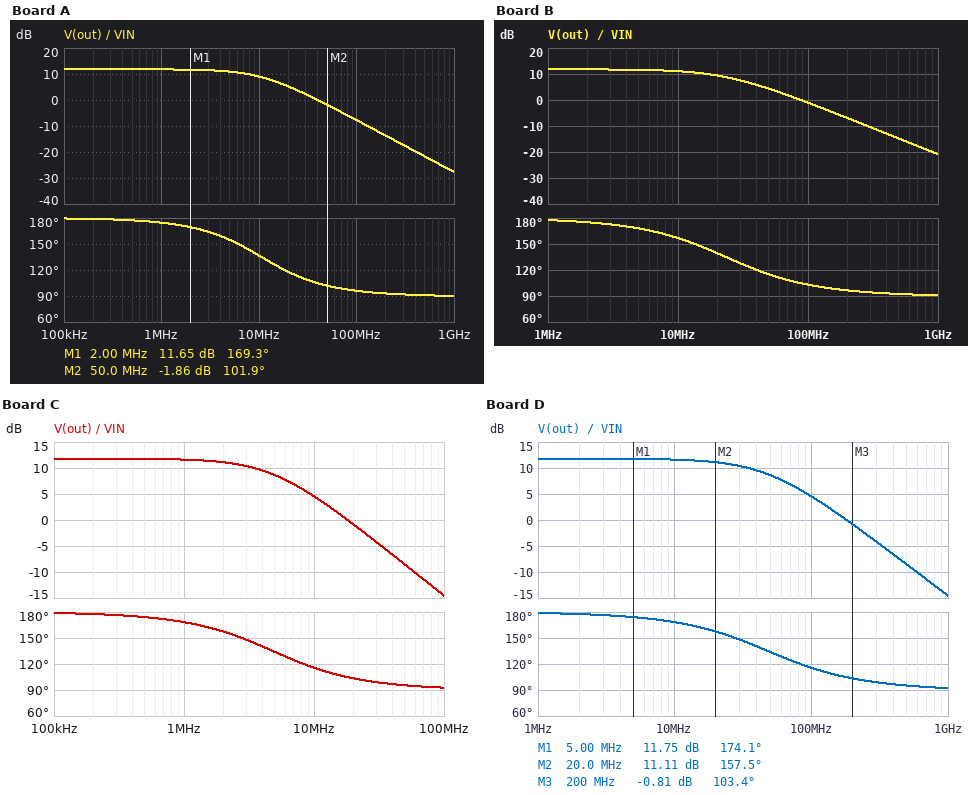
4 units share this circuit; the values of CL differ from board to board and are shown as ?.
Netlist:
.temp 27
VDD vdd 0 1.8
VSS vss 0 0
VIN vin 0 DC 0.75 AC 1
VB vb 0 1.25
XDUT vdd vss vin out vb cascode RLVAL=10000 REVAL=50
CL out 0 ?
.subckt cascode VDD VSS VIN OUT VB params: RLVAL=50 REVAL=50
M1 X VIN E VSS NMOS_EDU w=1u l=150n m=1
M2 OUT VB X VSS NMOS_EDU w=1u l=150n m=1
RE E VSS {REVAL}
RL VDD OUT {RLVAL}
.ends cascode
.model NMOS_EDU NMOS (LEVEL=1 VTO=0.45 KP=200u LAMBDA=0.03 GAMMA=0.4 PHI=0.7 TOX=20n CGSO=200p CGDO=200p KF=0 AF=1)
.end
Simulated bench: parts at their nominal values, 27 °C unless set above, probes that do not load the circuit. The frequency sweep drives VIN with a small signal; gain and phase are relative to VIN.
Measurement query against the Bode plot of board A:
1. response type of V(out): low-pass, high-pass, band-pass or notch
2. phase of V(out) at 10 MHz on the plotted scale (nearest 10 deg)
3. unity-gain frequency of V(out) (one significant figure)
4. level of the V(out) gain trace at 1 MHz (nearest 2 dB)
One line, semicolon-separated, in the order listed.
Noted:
low-pass; 140 deg; 40 MHz; 12 dB
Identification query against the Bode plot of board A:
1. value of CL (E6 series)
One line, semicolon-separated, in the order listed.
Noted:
1.5 pF
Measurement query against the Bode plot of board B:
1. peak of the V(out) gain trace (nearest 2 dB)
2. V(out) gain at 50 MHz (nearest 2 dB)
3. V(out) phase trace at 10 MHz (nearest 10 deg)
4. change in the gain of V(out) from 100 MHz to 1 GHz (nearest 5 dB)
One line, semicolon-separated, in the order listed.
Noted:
12 dB; 4 dB; 160 deg; -20 dB
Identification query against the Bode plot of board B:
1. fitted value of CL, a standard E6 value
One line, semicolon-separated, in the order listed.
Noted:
680 fF
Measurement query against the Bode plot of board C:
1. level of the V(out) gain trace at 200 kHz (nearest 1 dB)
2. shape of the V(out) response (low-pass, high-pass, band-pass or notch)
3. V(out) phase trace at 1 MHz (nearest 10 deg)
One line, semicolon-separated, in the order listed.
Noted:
12 dB; low-pass; 170 deg
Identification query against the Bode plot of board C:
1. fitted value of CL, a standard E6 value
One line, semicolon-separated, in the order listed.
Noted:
3.3 pF
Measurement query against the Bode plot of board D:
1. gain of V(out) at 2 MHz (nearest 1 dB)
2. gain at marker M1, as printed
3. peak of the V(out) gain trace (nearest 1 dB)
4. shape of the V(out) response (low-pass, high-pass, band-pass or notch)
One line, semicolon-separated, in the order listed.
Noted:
12 dB; 11.75 dB; 12 dB; low-pass
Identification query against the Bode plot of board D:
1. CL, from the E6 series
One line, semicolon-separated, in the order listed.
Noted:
330 fF
